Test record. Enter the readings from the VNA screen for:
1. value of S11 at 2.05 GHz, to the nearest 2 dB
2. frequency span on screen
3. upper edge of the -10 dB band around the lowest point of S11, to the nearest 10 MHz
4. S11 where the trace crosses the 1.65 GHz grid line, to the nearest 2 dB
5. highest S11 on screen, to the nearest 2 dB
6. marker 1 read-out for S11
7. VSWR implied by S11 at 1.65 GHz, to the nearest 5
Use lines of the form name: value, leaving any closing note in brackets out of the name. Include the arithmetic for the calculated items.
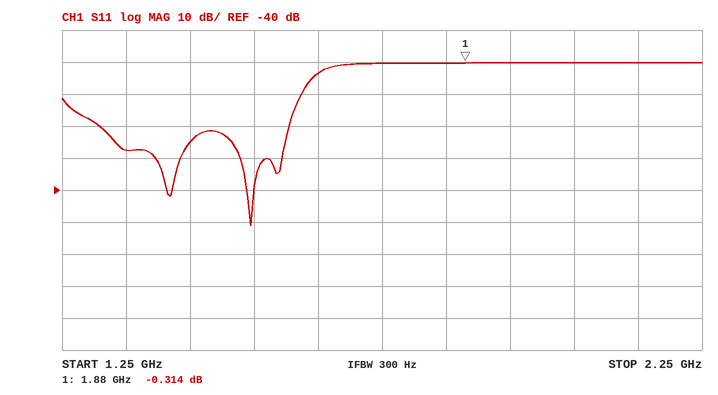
value of S11 at 2.05 GHz, to the nearest 2 dB: 0 dB
frequency span on screen: 1 GHz
upper edge of the -10 dB band around the lowest point of S11, to the nearest 10 MHz: 1.62 GHz
S11 where the trace crosses the 1.65 GHz grid line, to the nearest 2 dB: -4 dB
highest S11 on screen, to the nearest 2 dB: 0 dB
marker 1 read-out for S11: -0.314 dB
VSWR implied by S11 at 1.65 GHz, to the nearest 5: |Γ| = 10^(-4/20) = 0.6310; VSWR = (1 + 0.6310)/(1 − 0.6310) ≈ 4.42, so 5 to the nearest 5
